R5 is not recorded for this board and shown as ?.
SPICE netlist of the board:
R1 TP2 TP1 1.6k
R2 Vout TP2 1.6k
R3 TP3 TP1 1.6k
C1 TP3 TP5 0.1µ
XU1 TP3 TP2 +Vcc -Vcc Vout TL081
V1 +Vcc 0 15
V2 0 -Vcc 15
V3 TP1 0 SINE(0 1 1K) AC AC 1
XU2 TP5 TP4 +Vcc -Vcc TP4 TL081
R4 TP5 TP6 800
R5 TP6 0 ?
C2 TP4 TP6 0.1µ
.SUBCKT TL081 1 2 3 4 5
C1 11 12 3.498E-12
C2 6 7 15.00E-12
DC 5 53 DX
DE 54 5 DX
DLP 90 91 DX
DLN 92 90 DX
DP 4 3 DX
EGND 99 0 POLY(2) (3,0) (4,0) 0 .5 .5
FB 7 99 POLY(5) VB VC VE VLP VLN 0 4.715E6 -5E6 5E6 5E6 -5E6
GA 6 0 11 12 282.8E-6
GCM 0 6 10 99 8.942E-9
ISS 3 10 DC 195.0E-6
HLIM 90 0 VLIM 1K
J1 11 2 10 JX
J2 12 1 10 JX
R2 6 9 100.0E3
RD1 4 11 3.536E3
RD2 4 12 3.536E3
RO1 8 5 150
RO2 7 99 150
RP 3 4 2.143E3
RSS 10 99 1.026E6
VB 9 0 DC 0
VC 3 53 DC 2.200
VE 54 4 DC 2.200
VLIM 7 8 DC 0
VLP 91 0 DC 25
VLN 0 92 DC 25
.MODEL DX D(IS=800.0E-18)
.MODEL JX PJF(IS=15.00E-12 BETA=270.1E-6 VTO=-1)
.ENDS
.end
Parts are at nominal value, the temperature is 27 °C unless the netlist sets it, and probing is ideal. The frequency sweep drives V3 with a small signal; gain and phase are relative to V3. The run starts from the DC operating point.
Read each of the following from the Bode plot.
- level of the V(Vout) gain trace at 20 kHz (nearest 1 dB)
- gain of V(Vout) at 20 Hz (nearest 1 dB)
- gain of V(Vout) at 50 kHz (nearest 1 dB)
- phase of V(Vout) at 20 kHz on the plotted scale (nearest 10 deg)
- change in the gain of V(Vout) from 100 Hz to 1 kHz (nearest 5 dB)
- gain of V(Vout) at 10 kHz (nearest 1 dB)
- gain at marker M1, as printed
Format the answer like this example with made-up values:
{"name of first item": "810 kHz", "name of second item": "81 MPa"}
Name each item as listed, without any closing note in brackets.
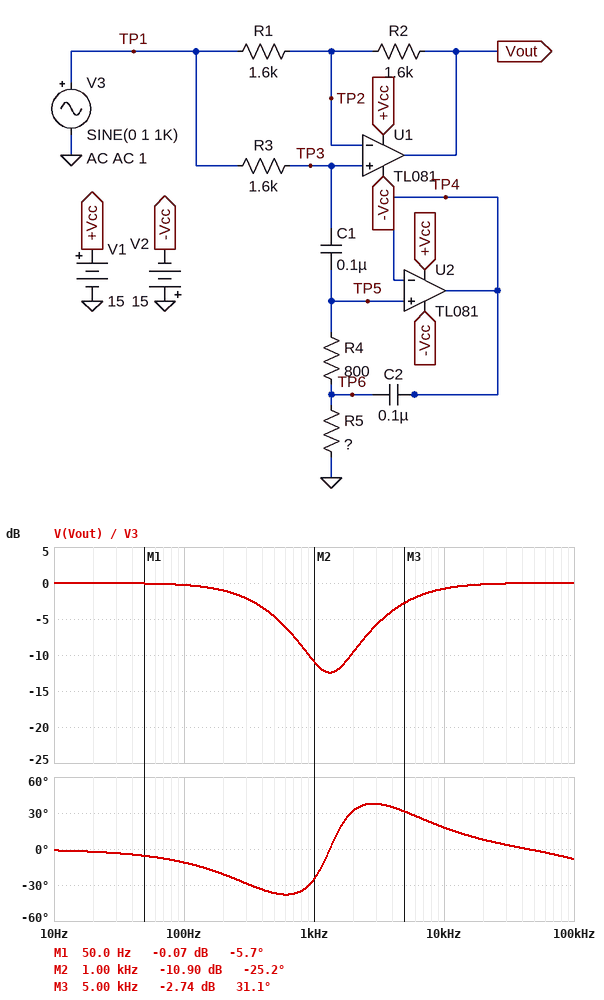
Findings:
{"level of the V(Vout) gain trace at 20 kHz": "0 dB", "gain of V(Vout) at 20 Hz": "0 dB", "gain of V(Vout) at 50 kHz": "0 dB", "phase of V(Vout) at 20 kHz on the plotted scale": "10 deg", "change in the gain of V(Vout) from 100 Hz to 1 kHz": "-10 dB", "gain of V(Vout) at 10 kHz": "-1 dB", "gain at marker M1, as printed": "-0.07 dB"}
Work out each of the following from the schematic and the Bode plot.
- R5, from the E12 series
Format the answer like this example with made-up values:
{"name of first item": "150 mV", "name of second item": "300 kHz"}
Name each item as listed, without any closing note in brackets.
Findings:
{"R5, from the E12 series": "1.8 kΩ"}
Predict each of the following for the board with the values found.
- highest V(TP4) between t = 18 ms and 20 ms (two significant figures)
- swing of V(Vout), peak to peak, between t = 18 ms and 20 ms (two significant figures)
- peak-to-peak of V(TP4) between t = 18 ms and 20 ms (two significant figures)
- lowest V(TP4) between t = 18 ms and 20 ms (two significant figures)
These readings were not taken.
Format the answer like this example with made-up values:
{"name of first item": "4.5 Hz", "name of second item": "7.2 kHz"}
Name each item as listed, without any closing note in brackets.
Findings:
{"highest V(TP4) between t = 18 ms and 20 ms": "650 mV", "swing of V(Vout), peak to peak, between t = 18 ms and 20 ms": "570 mV", "peak-to-peak of V(TP4) between t = 18 ms and 20 ms": "1.3 V", "lowest V(TP4) between t = 18 ms and 20 ms": "-650 mV"}
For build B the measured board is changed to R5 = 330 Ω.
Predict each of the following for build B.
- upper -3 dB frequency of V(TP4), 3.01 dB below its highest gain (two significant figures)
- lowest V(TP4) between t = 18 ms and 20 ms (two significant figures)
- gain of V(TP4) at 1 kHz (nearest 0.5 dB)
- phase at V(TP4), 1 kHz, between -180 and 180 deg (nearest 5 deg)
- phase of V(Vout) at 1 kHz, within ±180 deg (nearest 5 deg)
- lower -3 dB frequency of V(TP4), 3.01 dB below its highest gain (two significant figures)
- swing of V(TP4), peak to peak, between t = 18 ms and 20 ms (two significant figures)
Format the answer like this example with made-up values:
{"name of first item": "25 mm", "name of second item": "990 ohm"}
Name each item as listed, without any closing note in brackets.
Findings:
{"upper -3 dB frequency of V(TP4), 3.01 dB below its highest gain": "860 kHz", "lowest V(TP4) between t = 18 ms and 20 ms": "-370 mV", "gain of V(TP4) at 1 kHz": "-8.5 dB", "phase at V(TP4), 1 kHz, between -180 and 180 deg": "35 deg", "phase of V(Vout) at 1 kHz, within ±180 deg": "-80 deg", "lower -3 dB frequency of V(TP4), 3.01 dB below its highest gain": "12 kHz", "swing of V(TP4), peak to peak, between t = 18 ms and 20 ms": "740 mV"}
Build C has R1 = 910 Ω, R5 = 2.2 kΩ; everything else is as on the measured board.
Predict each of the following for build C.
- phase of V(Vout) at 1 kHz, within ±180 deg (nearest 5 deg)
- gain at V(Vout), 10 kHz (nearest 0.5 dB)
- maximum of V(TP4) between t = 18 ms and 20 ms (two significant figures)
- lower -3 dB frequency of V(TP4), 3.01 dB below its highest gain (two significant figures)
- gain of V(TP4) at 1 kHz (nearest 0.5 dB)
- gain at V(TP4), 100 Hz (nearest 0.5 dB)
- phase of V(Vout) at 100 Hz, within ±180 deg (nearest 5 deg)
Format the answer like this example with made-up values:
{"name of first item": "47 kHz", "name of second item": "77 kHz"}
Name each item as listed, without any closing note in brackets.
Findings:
{"phase of V(Vout) at 1 kHz, within ±180 deg": "-65 deg", "gain at V(Vout), 10 kHz": "-0.5 dB", "maximum of V(TP4) between t = 18 ms and 20 ms": "690 mV", "lower -3 dB frequency of V(TP4), 3.01 dB below its highest gain": "1.1 kHz", "gain of V(TP4) at 1 kHz": "-3.0 dB", "gain at V(TP4), 100 Hz": "-15.0 dB", "phase of V(Vout) at 100 Hz, within ±180 deg": "-15 deg"}
